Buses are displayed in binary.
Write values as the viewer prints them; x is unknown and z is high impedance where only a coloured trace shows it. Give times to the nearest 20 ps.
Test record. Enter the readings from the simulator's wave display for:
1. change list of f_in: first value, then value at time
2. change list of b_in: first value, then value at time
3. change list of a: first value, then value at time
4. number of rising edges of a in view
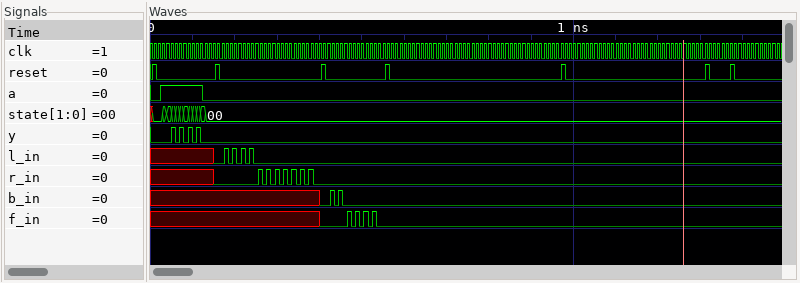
x, 0 at 400 ps, 1 at 460 ps, 0 at 480 ps, 1 at 480 ps, 0 at 500 ps, 1 at 500 ps, 0 at 520 ps, 1 at 520 ps, 0 at 540 ps
x, 0 at 400 ps, 1 at 420 ps, 0 at 440 ps, 1 at 440 ps, 0 at 460 ps
0, 1 at 20 ps, 0 at 120 ps
1
